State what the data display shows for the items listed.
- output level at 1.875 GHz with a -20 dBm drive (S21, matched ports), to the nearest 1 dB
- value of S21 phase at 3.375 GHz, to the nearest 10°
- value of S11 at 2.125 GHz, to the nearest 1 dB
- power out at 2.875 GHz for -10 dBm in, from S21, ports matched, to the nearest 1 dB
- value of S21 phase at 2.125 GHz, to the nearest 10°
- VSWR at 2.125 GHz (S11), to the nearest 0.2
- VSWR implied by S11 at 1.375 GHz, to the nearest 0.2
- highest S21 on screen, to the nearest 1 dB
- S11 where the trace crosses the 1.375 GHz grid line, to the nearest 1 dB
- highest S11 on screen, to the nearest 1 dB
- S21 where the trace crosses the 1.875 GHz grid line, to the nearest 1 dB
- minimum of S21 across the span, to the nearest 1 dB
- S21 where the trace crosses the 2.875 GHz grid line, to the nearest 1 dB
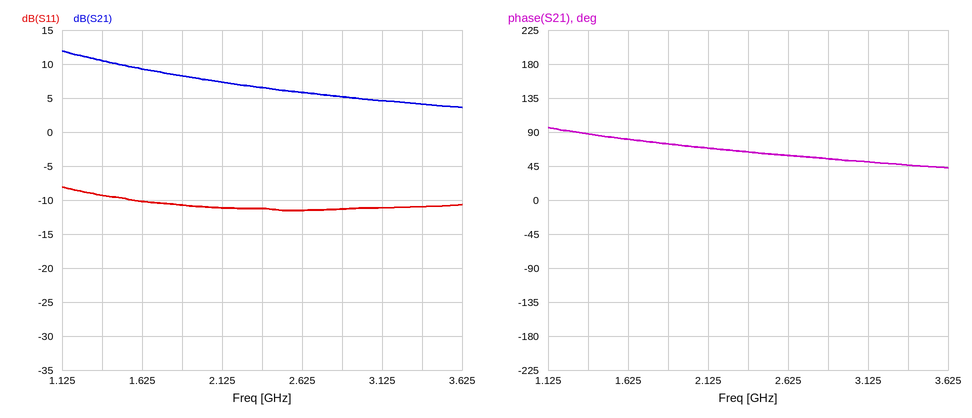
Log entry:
-12 dBm
50°
-11 dB
-5 dBm
70°
1.8
2.0
12 dB
-9 dB
-8 dB
8 dB
4 dB
5 dB
